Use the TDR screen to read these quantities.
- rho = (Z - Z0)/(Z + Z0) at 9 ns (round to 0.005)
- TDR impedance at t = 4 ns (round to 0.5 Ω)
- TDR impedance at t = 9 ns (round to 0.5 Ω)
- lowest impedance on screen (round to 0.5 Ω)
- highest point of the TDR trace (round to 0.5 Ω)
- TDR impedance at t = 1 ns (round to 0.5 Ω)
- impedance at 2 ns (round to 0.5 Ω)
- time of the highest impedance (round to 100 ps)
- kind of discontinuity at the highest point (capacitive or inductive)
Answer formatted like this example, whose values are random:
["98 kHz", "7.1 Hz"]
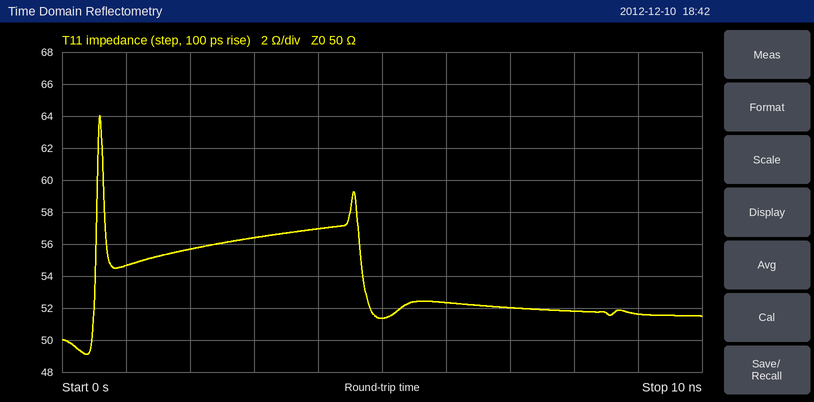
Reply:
["+0.015", "57.0 Ω", "51.5 Ω", "49.0 Ω", "64.0 Ω", "54.5 Ω", "55.5 Ω", "600 ps", "inductive"]
